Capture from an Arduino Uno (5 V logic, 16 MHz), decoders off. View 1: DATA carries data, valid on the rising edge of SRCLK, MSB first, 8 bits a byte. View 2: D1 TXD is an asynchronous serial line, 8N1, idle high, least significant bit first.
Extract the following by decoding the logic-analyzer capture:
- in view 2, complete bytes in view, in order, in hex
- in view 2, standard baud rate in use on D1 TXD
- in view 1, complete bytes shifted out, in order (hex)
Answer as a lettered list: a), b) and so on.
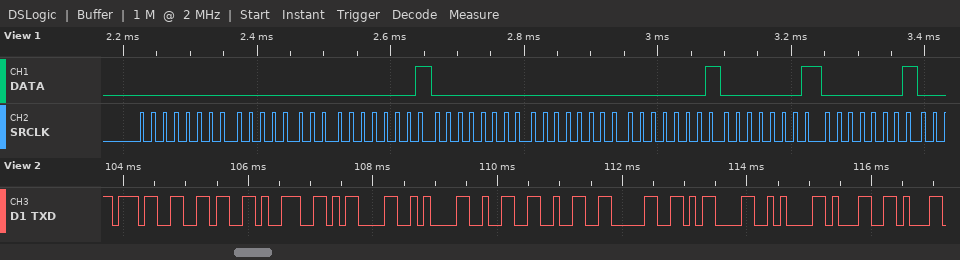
a) 37 36 39 0D 0A 32 32 30 0D 0A 31
b) 9600 baud
c) 00 00 01 00 00 01 01 01
